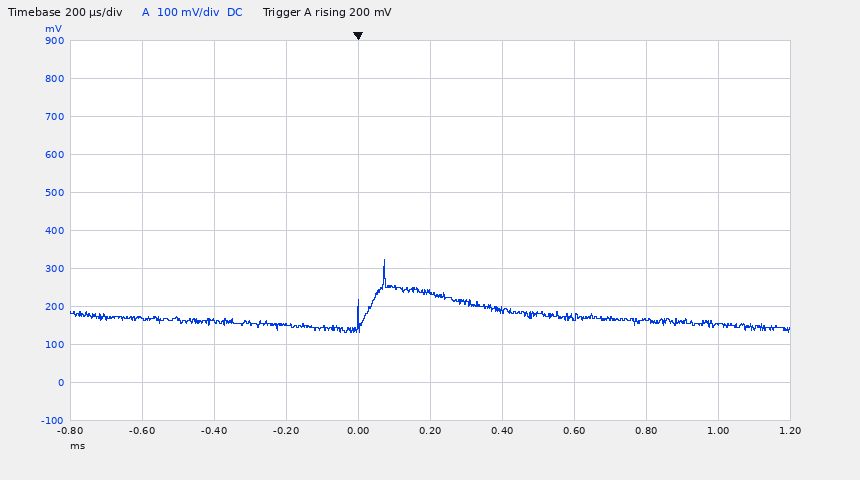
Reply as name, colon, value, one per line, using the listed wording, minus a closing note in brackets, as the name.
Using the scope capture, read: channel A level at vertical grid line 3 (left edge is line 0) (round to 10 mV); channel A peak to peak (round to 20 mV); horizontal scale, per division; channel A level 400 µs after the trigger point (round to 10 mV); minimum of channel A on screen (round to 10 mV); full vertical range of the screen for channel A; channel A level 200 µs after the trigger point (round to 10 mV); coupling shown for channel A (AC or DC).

channel A level at vertical grid line 3 (left edge is line 0): 150 mV
channel A peak to peak: 200 mV
horizontal scale, per division: 200 µs
channel A level 400 µs after the trigger point: 190 mV
minimum of channel A on screen: 130 mV
full vertical range of the screen for channel A: 1 V
channel A level 200 µs after the trigger point: 240 mV
coupling shown for channel A: DC
